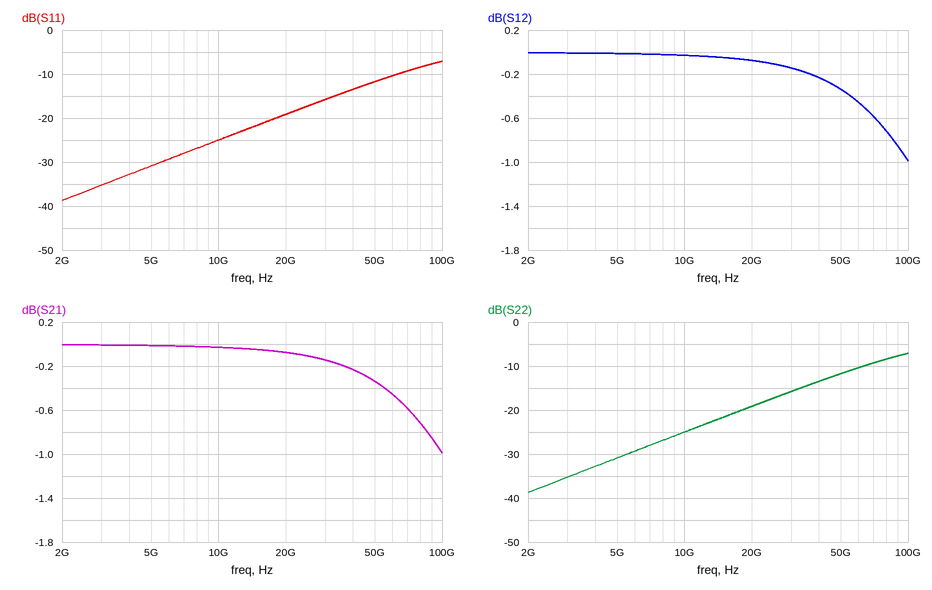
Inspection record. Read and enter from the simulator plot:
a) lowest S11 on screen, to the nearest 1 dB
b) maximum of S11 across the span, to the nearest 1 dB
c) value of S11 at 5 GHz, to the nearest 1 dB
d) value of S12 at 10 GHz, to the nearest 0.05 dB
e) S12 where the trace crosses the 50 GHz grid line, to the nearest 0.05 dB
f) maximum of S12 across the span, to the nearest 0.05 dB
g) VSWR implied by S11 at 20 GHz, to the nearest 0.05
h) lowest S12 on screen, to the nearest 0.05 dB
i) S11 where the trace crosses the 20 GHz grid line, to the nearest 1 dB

-39 dB
-7 dB
-31 dB
-0.05 dB
-0.35 dB
0.00 dB
1.25
-1.00 dB
-19 dB
